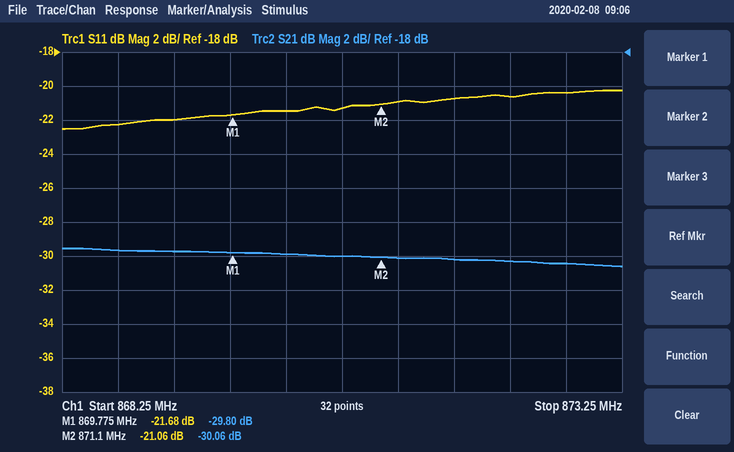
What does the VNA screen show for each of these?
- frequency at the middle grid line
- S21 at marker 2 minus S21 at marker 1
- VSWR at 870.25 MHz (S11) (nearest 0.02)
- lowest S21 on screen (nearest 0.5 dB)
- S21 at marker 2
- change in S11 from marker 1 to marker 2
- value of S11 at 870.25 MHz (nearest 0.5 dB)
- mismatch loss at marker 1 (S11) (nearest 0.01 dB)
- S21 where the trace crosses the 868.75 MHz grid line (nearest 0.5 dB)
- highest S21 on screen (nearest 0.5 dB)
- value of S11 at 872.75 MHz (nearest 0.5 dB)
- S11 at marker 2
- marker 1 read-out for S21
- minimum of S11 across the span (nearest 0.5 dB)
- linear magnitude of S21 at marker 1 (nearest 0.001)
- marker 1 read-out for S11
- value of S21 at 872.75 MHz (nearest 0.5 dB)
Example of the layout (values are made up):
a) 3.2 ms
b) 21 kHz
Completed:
a) 870.75 MHz
b) -0.26 dB
c) 1.18
d) -30.5 dB
e) -30.06 dB
f) 0.62 dB
g) -21.5 dB
h) 0.03 dB
i) -29.5 dB
j) -29.5 dB
k) -20.5 dB
l) -21.06 dB
m) -29.80 dB
n) -22.5 dB
o) 0.032
p) -21.68 dB
q) -30.5 dB
